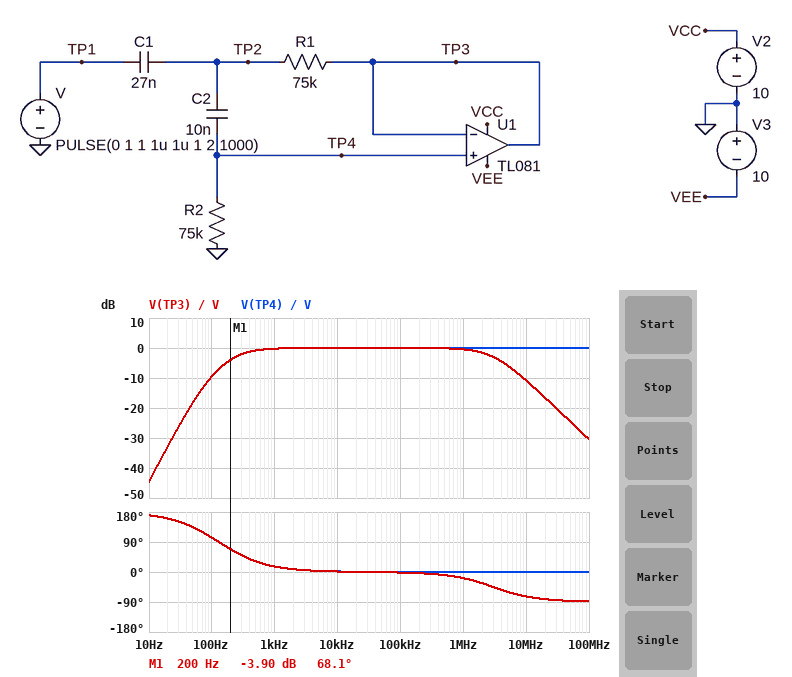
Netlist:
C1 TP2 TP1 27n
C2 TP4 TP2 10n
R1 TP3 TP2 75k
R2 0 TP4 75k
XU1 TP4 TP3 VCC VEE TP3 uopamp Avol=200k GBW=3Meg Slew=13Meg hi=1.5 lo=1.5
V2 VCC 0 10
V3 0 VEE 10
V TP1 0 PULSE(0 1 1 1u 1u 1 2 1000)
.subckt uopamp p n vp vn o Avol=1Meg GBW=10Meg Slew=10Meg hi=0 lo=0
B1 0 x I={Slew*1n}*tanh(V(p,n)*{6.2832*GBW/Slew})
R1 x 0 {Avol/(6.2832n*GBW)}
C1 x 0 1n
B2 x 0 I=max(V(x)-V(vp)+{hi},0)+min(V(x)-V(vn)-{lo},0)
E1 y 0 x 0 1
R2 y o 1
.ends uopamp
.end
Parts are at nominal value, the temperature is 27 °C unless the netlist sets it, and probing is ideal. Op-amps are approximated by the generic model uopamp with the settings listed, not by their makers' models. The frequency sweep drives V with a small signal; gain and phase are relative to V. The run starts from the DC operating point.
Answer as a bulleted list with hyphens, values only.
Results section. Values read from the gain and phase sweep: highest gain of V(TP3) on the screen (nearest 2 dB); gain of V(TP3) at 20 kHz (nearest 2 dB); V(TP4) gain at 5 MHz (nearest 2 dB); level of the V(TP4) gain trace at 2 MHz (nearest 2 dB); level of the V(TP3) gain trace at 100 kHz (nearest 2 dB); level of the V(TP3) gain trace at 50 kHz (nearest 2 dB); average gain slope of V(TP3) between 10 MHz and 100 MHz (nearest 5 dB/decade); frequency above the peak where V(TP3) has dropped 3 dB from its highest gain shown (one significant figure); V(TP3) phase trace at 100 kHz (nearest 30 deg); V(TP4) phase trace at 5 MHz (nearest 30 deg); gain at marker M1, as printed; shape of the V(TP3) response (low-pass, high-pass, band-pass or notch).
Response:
- 0 dB
- 0 dB
- 0 dB
- 0 dB
- 0 dB
- 0 dB
- -20 dB/decade
- 3 MHz
- 0 deg
- 0 deg
- -3.90 dB
- band-pass
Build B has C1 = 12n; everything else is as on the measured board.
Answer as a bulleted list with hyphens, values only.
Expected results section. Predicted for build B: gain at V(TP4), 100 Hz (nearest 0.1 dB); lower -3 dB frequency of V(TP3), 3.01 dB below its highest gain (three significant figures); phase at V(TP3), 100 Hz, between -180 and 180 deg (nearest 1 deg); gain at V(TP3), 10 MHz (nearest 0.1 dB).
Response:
- -13.6 dB
- 303 Hz
- 125 deg
- -10.8 dB
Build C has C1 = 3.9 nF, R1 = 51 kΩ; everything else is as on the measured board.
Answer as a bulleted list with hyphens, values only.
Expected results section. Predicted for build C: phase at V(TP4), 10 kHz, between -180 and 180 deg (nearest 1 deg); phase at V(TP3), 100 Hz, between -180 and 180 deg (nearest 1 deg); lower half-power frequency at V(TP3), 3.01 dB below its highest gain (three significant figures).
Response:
- 4 deg
- 155 deg
- 567 Hz
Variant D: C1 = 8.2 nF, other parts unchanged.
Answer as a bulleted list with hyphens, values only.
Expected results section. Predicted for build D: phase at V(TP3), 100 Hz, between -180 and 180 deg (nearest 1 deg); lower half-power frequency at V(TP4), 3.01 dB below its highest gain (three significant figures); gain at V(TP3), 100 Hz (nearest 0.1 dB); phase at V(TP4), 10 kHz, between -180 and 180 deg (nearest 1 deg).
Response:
- 134 deg
- 367 Hz
- -16.3 dB
- 3 deg
